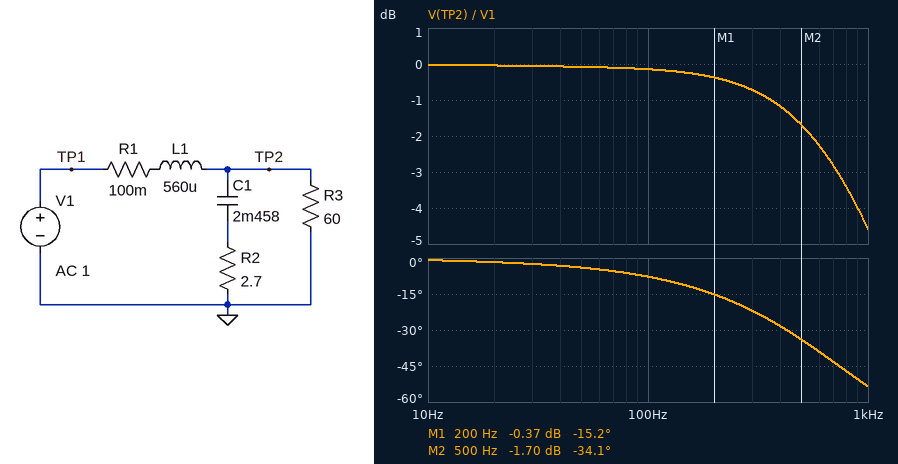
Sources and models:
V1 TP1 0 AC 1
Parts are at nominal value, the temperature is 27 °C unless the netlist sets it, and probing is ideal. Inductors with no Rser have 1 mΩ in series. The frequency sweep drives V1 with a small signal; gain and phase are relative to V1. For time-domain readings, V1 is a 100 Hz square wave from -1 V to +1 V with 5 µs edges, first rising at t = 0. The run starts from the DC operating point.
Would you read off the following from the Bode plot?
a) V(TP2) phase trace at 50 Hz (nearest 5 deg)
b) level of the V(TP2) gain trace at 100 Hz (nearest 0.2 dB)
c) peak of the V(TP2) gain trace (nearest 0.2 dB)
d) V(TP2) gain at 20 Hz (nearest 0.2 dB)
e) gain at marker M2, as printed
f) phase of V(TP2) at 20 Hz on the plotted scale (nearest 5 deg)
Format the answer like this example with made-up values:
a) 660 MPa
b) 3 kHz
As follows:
a) -5 deg
b) -0.2 dB
c) 0 dB
d) 0 dB
e) -1.70 dB
f) 0 deg
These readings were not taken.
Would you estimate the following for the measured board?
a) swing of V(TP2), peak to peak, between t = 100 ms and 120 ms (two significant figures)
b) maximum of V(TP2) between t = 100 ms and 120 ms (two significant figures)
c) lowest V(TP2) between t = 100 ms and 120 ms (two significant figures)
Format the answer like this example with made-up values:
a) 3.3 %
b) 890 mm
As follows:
a) 2.0 V
b) 990 mV
c) -990 mV
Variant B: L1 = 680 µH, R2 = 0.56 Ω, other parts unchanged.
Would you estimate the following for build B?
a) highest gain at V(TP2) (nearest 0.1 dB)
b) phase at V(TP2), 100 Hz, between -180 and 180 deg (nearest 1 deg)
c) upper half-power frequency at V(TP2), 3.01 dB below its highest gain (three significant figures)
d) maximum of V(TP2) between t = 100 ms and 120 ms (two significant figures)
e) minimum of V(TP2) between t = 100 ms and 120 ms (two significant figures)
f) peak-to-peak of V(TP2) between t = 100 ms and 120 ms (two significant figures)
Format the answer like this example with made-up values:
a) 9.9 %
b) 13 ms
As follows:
a) 1.8 dB
b) -31 deg
c) 176 Hz
d) 1.4 V
e) -1.4 V
f) 2.8 V
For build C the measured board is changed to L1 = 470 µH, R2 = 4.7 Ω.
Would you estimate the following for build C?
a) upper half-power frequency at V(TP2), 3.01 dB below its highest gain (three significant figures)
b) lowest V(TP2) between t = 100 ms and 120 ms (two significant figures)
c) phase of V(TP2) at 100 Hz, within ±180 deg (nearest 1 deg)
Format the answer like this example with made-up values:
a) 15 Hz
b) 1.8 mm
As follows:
a) 1.46 kHz
b) -990 mV
c) -4 deg
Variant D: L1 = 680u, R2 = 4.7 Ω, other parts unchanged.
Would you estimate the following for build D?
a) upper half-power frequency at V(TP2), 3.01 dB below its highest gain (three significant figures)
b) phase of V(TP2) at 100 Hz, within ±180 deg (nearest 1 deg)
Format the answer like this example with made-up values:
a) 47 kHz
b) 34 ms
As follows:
a) 1.01 kHz
b) -6 deg
